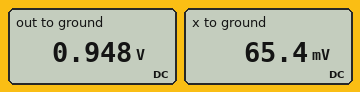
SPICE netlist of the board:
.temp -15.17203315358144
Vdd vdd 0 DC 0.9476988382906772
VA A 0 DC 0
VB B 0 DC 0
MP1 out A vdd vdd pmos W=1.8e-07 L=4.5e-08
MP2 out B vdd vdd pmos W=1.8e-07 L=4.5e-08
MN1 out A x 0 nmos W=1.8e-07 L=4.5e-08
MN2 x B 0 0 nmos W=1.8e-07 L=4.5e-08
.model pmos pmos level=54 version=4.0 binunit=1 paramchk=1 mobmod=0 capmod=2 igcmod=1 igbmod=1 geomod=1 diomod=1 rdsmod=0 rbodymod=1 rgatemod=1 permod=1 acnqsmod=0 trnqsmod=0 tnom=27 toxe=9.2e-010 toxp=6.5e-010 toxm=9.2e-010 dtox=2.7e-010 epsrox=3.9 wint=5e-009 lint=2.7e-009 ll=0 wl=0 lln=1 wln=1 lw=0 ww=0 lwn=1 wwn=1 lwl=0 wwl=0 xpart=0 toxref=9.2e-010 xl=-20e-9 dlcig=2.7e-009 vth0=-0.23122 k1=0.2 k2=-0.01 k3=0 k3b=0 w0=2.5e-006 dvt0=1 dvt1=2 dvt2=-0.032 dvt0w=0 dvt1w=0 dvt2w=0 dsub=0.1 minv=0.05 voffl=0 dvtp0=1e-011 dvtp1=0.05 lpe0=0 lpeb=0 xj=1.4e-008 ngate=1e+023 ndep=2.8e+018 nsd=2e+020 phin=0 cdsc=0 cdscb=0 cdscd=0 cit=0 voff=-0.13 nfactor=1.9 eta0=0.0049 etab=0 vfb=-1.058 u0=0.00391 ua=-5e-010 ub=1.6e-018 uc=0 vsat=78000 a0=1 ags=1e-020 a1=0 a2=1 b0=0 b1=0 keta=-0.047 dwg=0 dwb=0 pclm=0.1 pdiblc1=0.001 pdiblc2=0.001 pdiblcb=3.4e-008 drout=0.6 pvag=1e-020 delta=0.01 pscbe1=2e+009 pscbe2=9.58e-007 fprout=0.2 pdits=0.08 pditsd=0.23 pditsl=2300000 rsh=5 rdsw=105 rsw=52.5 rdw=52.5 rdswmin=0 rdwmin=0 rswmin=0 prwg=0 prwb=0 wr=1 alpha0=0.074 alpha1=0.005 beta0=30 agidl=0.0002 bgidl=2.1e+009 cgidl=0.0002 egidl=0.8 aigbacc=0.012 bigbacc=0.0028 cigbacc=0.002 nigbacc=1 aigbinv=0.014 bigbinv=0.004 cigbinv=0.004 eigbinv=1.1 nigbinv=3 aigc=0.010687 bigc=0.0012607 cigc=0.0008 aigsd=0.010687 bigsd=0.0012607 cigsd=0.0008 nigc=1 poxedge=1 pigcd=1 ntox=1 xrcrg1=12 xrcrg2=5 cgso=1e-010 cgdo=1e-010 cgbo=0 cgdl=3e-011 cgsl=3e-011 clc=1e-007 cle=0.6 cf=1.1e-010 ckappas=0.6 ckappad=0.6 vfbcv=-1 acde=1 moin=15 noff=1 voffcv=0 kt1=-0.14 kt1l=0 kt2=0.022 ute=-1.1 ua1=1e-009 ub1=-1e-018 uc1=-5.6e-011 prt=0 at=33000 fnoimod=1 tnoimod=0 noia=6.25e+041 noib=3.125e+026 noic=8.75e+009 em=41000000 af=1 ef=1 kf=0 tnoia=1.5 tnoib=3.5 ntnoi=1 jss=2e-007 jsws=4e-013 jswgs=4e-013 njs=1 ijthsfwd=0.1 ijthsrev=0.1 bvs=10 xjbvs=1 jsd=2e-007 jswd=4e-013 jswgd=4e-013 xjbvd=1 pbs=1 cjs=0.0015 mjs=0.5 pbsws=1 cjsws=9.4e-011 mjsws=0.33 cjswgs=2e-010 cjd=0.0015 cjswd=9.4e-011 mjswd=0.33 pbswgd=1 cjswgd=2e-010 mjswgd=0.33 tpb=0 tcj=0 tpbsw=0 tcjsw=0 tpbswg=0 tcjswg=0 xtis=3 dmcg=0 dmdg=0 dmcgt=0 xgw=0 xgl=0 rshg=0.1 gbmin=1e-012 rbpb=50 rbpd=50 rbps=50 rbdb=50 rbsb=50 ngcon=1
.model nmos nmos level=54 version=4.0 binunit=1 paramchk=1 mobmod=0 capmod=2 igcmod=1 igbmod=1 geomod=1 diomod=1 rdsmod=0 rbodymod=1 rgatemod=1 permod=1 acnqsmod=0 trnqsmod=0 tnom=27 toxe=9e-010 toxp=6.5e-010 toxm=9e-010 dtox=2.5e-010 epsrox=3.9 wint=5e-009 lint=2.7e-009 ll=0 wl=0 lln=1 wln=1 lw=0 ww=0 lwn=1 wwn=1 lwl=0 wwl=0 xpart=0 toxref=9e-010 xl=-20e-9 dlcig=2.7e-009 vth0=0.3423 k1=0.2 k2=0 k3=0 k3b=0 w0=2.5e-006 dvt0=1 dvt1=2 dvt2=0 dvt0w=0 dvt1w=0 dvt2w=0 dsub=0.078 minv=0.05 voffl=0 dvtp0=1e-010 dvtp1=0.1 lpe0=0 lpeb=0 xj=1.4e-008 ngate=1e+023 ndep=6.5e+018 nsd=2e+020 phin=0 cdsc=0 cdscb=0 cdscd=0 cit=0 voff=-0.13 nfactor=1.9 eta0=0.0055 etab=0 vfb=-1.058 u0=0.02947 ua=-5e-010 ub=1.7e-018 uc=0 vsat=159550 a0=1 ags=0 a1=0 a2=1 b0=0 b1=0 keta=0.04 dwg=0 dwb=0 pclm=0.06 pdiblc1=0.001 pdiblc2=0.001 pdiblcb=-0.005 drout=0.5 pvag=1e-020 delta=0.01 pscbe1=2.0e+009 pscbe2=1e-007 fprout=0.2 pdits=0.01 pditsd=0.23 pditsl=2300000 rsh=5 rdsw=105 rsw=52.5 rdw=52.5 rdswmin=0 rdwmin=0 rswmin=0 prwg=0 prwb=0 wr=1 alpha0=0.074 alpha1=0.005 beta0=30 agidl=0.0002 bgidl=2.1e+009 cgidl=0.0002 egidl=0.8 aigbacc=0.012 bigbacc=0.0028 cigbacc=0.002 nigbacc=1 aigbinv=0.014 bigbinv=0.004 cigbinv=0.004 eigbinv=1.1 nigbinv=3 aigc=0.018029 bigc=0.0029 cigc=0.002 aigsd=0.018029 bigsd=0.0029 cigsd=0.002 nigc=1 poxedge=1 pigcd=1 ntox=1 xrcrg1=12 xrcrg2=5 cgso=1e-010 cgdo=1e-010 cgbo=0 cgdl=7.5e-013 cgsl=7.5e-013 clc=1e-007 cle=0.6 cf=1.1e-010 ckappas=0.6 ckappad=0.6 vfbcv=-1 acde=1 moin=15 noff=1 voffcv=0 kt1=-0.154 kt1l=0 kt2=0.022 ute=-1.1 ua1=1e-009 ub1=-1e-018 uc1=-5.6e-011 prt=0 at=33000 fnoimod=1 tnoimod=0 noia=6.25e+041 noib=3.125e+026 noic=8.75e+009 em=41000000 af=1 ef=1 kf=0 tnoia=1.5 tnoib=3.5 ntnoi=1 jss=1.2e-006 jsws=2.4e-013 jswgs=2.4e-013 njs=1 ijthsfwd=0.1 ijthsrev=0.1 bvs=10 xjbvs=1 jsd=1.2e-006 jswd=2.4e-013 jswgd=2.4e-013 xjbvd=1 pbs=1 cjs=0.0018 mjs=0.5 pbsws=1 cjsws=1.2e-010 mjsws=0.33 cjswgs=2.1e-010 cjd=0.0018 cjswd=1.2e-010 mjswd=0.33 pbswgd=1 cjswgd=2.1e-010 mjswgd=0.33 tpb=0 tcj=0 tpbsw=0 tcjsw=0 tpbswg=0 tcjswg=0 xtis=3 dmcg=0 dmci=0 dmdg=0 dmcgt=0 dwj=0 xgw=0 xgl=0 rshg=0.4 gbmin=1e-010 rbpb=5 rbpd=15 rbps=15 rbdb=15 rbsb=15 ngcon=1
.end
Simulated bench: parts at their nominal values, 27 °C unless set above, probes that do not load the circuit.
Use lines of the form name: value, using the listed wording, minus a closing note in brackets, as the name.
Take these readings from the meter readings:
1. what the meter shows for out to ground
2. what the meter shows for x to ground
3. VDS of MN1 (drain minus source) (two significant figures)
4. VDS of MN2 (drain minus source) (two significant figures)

what the meter shows for out to ground: 0.948 V
what the meter shows for x to ground: 65.4 mV
VDS of MN1 (drain minus source): 880 mV
VDS of MN2 (drain minus source): 65 mV
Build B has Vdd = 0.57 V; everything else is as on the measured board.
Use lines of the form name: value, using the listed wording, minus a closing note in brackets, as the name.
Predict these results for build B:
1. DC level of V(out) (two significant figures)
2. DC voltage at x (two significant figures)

DC level of V(out): 570 mV
DC voltage at x: 42 mV
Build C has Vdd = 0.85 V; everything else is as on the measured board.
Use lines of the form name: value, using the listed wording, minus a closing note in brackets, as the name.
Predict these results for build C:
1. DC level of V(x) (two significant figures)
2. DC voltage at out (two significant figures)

DC level of V(x): 59 mV
DC voltage at out: 850 mV
